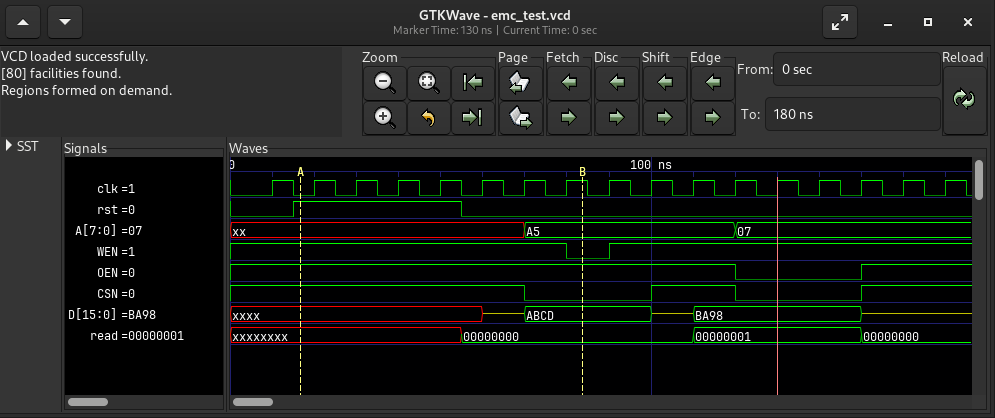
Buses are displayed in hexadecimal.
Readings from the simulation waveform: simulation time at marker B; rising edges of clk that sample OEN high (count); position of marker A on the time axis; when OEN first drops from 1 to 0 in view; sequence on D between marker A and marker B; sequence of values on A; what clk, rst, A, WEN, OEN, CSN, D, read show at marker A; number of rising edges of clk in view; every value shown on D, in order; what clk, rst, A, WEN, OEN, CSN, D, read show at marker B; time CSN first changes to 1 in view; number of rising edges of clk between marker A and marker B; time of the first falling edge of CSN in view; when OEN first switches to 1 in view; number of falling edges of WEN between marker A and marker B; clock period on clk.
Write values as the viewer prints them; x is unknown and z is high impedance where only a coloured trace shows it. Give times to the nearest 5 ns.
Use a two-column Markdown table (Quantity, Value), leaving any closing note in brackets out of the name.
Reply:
| Quantity | Value |
|---|---|
| simulation time at marker B | 85 ns |
| rising edges of clk that sample OEN high | 14 |
| position of marker A on the time axis | 15 ns |
| when OEN first drops from 1 to 0 in view | 120 ns |
| sequence on D between marker A and marker B | xxxx, z, ABCD |
| sequence of values on A | xx, A5, 07 |
| what clk, rst, A, WEN, OEN, CSN, D, read show at marker A | clk=0, rst=1, A=xx, WEN=1, OEN=1, CSN=1, D=xxxx, read=xxxxxxxx |
| number of rising edges of clk in view | 17 |
| every value shown on D, in order | xxxx, z, ABCD, z, BA98, z |
| what clk, rst, A, WEN, OEN, CSN, D, read show at marker B | clk=1, rst=0, A=A5, WEN=0, OEN=1, CSN=0, D=ABCD, read=00000000 |
| time CSN first changes to 1 in view | 100 ns |
| number of rising edges of clk between marker A and marker B | 7 |
| time of the first falling edge of CSN in view | 70 ns |
| when OEN first switches to 1 in view | 150 ns |
| number of falling edges of WEN between marker A and marker B | 1 |
| clock period on clk | 10 ns |
